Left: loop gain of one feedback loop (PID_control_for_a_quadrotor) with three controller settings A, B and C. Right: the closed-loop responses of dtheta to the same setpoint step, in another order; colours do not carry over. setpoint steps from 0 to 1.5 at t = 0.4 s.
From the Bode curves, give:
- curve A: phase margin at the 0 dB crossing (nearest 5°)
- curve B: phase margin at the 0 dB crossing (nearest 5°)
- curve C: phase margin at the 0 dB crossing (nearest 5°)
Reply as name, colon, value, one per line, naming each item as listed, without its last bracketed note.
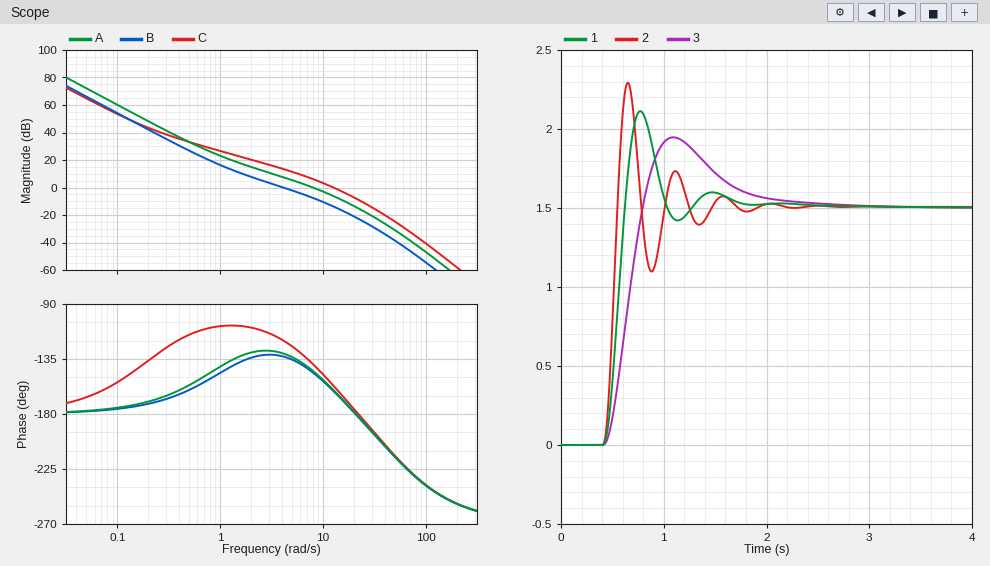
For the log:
curve A: phase margin at the 0 dB crossing: 35°
curve B: phase margin at the 0 dB crossing: 45°
curve C: phase margin at the 0 dB crossing: 25°
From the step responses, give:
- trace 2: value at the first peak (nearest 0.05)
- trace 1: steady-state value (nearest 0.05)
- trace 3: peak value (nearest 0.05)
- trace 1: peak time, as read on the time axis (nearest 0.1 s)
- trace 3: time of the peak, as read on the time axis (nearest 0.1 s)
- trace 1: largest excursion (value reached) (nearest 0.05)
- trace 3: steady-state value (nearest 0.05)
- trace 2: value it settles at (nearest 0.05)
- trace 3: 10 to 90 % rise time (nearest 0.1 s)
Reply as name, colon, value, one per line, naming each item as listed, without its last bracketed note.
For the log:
trace 2: value at the first peak: 2.30
trace 1: steady-state value: 1.50
trace 3: peak value: 1.95
trace 1: peak time, as read on the time axis: 0.8 s
trace 3: time of the peak, as read on the time axis: 1.1 s
trace 1: largest excursion (value reached): 2.10
trace 3: steady-state value: 1.50
trace 2: value it settles at: 1.50
trace 3: 10 to 90 % rise time: 0.3 s
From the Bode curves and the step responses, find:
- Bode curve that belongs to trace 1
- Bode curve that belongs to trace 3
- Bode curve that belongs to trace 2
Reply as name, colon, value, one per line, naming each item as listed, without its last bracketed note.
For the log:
Bode curve that belongs to trace 1: A
Bode curve that belongs to trace 3: B
Bode curve that belongs to trace 2: C
